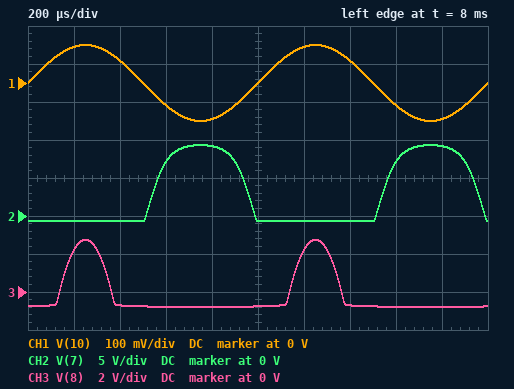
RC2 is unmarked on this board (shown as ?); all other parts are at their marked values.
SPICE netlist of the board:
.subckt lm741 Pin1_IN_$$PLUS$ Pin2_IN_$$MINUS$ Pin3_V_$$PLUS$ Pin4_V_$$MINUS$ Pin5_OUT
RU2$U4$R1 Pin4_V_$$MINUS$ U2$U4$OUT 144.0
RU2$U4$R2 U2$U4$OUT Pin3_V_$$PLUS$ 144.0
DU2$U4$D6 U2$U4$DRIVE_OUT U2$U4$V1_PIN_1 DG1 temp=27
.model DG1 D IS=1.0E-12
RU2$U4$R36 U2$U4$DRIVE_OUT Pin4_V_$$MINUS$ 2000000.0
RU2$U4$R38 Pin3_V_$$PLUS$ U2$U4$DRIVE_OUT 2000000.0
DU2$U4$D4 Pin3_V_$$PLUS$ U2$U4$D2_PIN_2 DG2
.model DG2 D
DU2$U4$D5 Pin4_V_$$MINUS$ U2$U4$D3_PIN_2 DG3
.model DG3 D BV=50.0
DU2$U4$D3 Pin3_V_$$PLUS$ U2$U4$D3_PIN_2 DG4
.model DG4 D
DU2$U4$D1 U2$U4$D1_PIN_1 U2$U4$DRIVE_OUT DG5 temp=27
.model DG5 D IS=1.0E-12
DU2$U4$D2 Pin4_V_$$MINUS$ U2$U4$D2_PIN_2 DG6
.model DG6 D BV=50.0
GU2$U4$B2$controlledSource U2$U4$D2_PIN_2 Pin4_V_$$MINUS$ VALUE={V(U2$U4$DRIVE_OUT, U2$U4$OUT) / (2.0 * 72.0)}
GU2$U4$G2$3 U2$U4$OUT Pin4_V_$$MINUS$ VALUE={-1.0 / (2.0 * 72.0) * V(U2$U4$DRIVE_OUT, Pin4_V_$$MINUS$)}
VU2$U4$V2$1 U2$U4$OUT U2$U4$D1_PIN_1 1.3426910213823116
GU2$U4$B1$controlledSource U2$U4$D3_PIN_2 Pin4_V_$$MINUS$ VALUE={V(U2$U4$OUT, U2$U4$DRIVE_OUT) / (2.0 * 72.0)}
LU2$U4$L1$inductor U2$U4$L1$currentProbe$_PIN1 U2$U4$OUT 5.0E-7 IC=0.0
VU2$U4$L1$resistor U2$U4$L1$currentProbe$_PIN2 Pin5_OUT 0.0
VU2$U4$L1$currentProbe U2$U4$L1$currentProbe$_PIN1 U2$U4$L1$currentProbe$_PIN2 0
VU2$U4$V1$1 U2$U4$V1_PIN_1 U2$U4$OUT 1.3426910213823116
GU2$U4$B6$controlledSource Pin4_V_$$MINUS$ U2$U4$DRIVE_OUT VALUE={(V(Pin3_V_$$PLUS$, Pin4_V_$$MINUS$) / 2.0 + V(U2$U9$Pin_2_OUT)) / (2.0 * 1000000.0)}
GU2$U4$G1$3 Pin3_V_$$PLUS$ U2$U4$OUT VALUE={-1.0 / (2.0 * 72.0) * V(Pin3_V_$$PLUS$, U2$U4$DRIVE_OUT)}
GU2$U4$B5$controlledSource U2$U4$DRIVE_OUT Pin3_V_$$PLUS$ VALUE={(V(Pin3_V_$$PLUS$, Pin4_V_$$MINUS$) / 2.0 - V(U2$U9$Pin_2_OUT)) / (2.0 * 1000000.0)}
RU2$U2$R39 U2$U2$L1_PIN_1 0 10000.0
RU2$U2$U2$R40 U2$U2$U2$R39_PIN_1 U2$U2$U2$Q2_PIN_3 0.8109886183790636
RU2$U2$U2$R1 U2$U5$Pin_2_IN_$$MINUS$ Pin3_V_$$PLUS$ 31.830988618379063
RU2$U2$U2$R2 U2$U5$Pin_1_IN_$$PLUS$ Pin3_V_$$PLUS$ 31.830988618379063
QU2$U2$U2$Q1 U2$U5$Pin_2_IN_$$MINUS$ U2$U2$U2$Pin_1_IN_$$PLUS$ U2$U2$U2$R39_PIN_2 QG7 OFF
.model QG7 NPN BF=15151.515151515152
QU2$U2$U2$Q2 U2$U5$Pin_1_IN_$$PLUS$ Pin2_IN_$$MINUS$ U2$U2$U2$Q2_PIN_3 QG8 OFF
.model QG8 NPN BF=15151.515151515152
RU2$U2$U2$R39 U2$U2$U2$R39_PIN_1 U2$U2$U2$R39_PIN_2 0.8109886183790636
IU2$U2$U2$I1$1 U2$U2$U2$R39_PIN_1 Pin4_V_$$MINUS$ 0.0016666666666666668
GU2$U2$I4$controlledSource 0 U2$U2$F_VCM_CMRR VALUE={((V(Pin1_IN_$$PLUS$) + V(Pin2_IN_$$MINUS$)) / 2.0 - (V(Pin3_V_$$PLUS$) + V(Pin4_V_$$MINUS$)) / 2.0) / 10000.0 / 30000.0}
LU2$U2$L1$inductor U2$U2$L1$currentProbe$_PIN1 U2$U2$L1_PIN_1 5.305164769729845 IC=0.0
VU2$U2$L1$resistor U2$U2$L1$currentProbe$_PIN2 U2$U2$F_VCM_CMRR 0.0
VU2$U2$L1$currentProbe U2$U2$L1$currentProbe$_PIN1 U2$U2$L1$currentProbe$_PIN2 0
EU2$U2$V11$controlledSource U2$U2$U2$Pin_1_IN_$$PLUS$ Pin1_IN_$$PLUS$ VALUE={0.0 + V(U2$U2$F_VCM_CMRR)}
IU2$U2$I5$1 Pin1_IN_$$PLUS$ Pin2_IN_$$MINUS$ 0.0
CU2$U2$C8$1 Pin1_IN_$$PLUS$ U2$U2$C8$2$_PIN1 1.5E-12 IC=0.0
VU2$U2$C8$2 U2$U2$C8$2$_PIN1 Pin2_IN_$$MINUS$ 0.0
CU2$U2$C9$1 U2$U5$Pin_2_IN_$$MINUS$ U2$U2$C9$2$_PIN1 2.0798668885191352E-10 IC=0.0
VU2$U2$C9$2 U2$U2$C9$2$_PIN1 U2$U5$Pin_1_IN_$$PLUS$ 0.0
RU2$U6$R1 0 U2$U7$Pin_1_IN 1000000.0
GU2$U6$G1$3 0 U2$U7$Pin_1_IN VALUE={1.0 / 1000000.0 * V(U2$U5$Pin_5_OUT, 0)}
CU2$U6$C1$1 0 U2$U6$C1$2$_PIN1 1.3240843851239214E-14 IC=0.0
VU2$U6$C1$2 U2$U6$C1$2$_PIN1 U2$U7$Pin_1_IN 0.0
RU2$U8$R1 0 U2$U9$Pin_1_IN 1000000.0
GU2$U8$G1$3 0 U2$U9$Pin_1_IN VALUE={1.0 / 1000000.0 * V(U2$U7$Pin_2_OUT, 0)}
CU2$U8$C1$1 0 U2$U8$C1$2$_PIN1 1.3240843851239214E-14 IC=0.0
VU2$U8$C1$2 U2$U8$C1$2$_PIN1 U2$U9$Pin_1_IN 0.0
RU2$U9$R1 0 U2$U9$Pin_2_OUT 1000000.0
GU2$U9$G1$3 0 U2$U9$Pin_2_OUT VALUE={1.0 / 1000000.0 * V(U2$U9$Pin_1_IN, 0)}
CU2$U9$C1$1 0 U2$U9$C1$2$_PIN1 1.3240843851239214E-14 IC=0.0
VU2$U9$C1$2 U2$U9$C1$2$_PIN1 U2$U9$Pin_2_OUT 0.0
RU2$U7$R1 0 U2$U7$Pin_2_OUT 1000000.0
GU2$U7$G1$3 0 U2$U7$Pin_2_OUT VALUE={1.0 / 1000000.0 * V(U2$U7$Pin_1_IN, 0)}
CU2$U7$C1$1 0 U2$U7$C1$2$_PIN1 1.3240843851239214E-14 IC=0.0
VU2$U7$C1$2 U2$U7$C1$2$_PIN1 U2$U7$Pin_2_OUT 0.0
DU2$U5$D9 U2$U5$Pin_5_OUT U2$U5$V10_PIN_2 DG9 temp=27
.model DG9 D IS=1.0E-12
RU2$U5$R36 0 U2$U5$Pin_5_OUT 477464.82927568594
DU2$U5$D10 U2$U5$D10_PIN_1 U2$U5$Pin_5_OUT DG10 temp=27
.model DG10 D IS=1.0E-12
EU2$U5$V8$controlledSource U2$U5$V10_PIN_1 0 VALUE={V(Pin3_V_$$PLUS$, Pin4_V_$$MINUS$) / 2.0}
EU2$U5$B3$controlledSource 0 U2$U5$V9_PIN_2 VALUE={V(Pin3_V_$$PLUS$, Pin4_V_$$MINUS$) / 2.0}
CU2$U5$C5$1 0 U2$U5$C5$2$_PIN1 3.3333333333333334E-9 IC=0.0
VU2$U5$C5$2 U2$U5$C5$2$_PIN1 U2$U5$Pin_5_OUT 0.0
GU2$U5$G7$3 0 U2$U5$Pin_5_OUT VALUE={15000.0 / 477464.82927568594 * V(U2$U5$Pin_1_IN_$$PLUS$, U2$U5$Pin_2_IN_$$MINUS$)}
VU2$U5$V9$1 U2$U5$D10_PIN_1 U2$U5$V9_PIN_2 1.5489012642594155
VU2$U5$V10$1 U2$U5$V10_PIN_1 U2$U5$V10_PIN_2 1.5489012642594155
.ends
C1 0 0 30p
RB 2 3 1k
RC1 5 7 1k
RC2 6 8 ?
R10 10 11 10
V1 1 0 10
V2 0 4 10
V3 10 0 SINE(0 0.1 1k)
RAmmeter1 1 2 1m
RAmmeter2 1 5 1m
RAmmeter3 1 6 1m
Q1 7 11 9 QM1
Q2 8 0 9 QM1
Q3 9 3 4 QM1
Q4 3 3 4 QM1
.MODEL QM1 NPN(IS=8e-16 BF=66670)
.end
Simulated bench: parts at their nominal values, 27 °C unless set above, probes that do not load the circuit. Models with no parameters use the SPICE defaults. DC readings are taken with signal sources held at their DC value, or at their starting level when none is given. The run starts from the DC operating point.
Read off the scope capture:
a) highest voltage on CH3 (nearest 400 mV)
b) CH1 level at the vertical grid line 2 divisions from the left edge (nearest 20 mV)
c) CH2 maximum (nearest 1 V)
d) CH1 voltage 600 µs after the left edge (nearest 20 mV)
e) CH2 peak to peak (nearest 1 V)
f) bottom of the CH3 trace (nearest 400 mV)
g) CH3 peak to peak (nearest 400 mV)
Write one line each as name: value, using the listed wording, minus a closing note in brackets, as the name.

highest voltage on CH3: 2.8 V
CH1 level at the vertical grid line 2 divisions from the left edge: 60 mV
CH2 maximum: 9 V
CH1 voltage 600 µs after the left edge: -60 mV
CH2 peak to peak: 10 V
bottom of the CH3 trace: -800 mV
CH3 peak to peak: 3.6 V
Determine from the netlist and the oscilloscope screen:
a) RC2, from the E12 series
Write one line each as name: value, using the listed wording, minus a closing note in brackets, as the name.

RC2, from the E12 series: 2.2 kΩ
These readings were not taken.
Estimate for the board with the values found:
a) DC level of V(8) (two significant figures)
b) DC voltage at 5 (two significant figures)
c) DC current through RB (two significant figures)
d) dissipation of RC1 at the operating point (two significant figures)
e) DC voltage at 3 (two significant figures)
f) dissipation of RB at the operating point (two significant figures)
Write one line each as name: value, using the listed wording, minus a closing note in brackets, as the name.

DC level of V(8): -750 mV
DC voltage at 5: 10 V
DC current through RB: 19 mA
dissipation of RC1 at the operating point: 110 mW
DC voltage at 3: -9.2 V
dissipation of RB at the operating point: 370 mW
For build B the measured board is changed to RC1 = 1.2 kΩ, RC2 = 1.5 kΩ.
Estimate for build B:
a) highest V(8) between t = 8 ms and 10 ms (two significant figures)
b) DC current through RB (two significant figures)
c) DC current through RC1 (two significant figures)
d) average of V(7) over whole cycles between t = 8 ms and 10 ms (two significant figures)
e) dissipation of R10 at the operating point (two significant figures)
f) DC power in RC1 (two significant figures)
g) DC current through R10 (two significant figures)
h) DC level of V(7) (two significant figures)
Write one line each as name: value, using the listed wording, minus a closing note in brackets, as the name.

highest V(8) between t = 8 ms and 10 ms: 3.5 V
DC current through RB: 19 mA
DC current through RC1: 8.9 mA
average of V(7) over whole cycles between t = 8 ms and 10 ms: 2.8 V
dissipation of R10 at the operating point: 2.9 µW
DC power in RC1: 96 mW
DC current through R10: 540 µA
DC level of V(7): -710 mV
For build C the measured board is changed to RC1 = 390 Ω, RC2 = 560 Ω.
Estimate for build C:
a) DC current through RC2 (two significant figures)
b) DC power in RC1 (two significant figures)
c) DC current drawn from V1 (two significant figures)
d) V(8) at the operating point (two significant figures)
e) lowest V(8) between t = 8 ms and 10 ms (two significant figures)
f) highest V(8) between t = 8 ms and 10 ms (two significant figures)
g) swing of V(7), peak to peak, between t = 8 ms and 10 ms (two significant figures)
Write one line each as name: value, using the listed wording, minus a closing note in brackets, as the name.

DC current through RC2: 9.6 mA
DC power in RC1: 36 mW
DC current drawn from V1: 38 mA
V(8) at the operating point: 4.6 V
lowest V(8) between t = 8 ms and 10 ms: -530 mV
highest V(8) between t = 8 ms and 10 ms: 9.8 V
swing of V(7), peak to peak, between t = 8 ms and 10 ms: 7.2 V
